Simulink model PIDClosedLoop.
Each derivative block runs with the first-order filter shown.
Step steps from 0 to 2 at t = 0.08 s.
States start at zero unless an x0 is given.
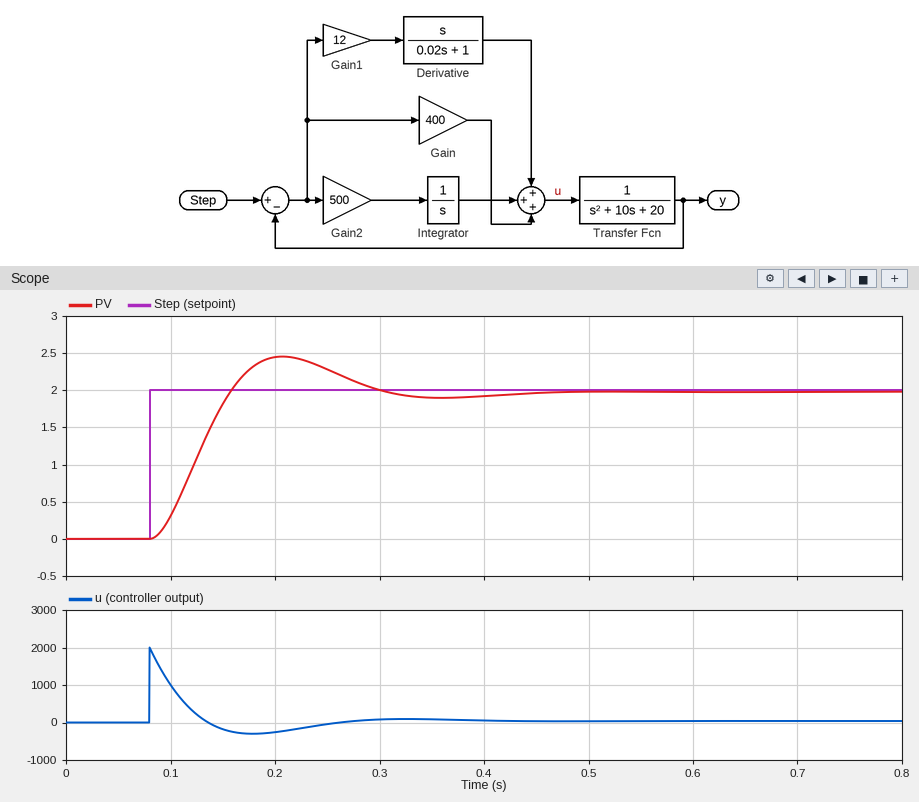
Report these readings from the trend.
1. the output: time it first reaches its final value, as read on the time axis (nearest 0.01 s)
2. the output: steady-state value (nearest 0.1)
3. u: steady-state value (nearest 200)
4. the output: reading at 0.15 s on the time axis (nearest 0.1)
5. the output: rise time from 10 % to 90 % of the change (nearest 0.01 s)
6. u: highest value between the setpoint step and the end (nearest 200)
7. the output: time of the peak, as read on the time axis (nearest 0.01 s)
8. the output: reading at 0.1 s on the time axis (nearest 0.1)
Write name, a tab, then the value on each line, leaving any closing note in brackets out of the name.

the output: time it first reaches its final value, as read on the time axis	0.16 s
the output: steady-state value	2.0
u: steady-state value	0
the output: reading at 0.15 s on the time axis	1.8
the output: rise time from 10 % to 90 % of the change	0.05 s
u: highest value between the setpoint step and the end	2000
the output: time of the peak, as read on the time axis	0.21 s
the output: reading at 0.1 s on the time axis	0.3
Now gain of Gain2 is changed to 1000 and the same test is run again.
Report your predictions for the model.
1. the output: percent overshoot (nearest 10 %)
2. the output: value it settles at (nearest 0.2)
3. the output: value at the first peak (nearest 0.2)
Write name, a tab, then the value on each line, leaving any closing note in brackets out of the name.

the output: percent overshoot	30 %
the output: value it settles at	2.0
the output: value at the first peak	2.6
